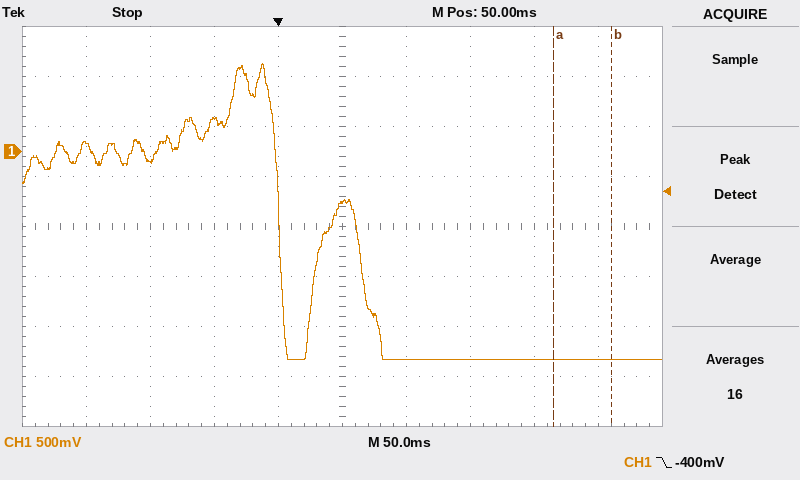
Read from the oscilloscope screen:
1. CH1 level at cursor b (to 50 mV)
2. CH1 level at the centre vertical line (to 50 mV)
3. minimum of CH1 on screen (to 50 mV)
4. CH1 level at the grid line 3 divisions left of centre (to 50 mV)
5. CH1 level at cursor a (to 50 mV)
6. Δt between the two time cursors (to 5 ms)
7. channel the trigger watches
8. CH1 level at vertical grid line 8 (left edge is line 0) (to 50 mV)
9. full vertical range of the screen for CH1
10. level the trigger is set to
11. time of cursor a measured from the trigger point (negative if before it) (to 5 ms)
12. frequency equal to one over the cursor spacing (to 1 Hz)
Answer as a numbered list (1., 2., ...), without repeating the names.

1. -2.10 V
2. -500 mV
3. -2.10 V
4. -100 mV
5. -2.10 V
6. 45 ms
7. CH1
8. -2.10 V
9. 4 V
10. -400 mV
11. +215 ms
12. 22 Hz
